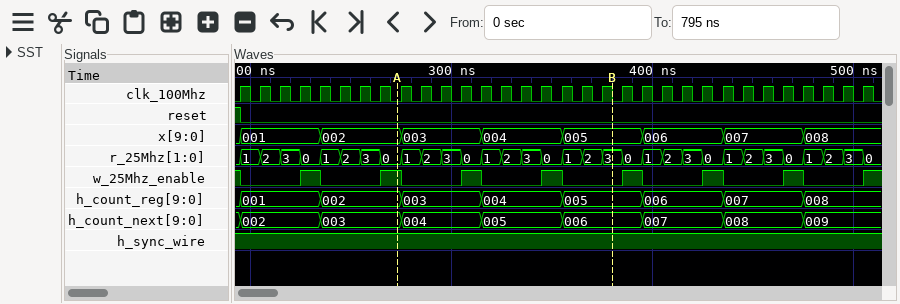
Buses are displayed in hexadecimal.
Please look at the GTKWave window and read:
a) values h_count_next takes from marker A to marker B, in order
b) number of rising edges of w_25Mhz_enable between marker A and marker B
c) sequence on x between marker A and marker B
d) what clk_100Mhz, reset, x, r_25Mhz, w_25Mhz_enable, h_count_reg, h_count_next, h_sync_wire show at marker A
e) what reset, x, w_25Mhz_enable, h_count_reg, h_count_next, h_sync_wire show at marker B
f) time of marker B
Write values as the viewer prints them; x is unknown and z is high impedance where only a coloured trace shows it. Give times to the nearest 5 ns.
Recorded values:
003, 004, 005, 006
2
002, 003, 004, 005
clk_100Mhz=0, reset=0, x=002, r_25Mhz=0, w_25Mhz_enable=1, h_count_reg=002, h_count_next=003, h_sync_wire=1
reset=0, x=005, w_25Mhz_enable=0, h_count_reg=005, h_count_next=006, h_sync_wire=1
380 ns
